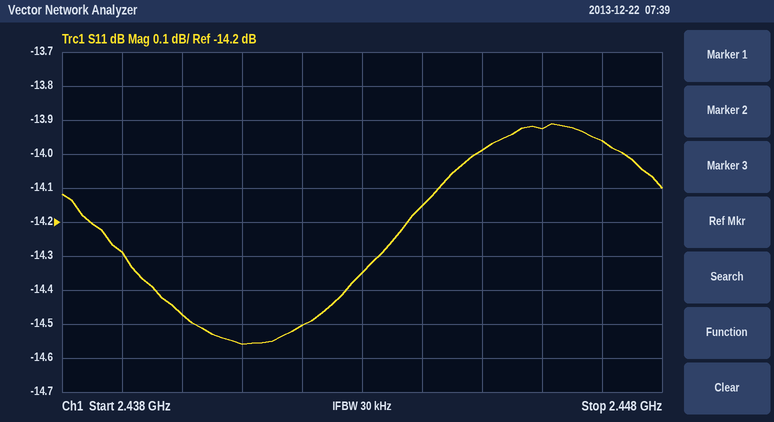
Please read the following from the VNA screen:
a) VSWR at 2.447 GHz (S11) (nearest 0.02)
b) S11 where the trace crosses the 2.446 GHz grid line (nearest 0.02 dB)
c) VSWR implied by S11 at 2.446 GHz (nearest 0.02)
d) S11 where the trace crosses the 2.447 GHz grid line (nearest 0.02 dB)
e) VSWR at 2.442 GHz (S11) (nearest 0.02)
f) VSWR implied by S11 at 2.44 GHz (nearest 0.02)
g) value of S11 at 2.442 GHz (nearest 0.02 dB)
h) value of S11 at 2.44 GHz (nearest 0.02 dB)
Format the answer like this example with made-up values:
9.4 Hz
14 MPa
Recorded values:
1.50
-13.92 dB
1.50
-13.96 dB
1.46
1.46
-14.50 dB
-14.48 dB
